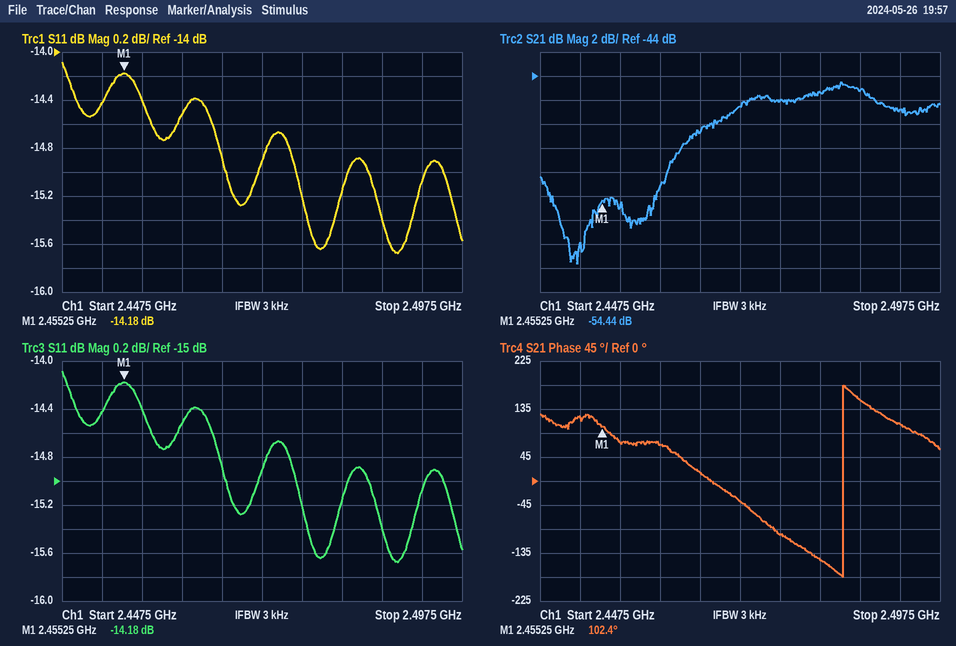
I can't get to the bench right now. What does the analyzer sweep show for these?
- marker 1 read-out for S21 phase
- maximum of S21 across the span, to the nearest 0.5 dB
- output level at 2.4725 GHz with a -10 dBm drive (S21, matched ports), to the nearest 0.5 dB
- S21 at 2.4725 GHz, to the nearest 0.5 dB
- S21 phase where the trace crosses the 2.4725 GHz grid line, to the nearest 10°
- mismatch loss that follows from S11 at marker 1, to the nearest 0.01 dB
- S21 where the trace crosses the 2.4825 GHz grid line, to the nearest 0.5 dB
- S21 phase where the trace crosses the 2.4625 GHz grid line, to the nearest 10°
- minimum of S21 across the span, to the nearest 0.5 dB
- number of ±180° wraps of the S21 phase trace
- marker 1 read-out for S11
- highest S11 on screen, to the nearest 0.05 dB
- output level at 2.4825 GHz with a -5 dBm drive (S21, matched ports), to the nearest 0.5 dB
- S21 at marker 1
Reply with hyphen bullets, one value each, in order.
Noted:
- 102.4°
- -44.5 dB
- -56.5 dBm
- -46.5 dB
- -40°
- 0.17 dB
- -45.5 dB
- 70°
- -59.5 dB
- 1
- -14.18 dB
- -14.10 dB
- -50.5 dBm
- -54.44 dB
